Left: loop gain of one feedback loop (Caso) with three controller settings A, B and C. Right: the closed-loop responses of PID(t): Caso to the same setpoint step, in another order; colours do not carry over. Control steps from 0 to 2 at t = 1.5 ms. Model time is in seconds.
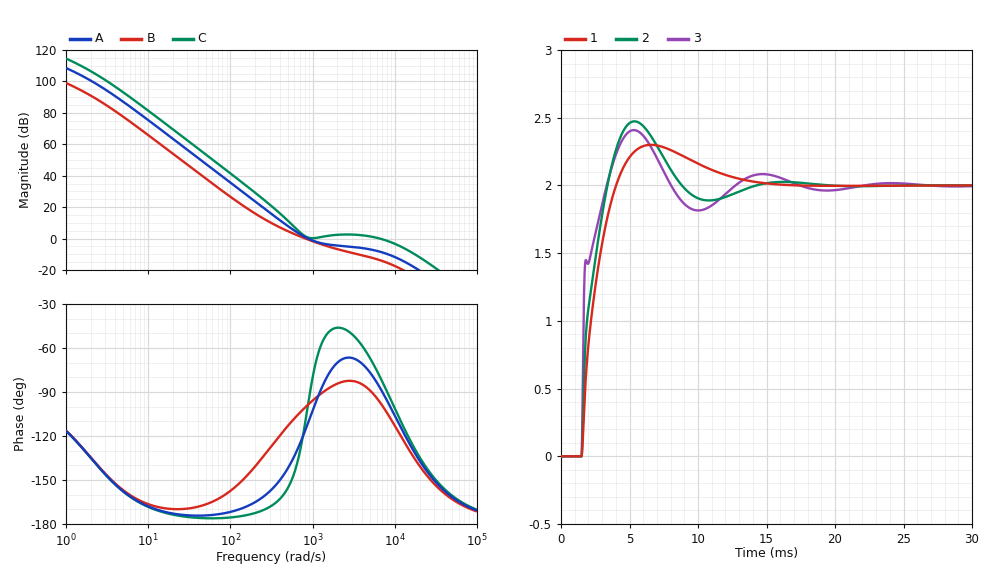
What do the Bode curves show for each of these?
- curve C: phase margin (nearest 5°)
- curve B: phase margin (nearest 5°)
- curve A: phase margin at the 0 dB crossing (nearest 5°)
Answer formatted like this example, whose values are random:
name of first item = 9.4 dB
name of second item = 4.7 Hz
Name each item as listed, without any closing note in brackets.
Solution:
curve C: phase margin = 100°
curve B: phase margin = 80°
curve A: phase margin at the 0 dB crossing = 70°
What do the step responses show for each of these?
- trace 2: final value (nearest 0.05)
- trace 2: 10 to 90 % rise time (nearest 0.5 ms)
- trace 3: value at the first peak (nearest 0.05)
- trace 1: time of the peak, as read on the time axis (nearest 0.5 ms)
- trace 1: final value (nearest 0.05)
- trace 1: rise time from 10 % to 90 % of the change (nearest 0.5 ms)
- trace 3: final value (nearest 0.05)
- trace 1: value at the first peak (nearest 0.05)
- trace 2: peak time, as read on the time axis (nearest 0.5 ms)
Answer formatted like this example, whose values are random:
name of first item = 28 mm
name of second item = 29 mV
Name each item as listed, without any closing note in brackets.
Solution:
trace 2: final value = 2.00
trace 2: 10 to 90 % rise time = 1.5 ms
trace 3: value at the first peak = 2.40
trace 1: time of the peak, as read on the time axis = 6.5 ms
trace 1: final value = 2.00
trace 1: rise time from 10 % to 90 % of the change = 2.0 ms
trace 3: final value = 2.00
trace 1: value at the first peak = 2.30
trace 2: peak time, as read on the time axis = 5.5 ms
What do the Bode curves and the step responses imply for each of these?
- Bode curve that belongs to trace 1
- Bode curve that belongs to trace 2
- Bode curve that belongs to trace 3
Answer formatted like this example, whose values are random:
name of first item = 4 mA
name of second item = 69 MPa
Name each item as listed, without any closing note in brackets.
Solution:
Bode curve that belongs to trace 1 = B
Bode curve that belongs to trace 2 = A
Bode curve that belongs to trace 3 = C
